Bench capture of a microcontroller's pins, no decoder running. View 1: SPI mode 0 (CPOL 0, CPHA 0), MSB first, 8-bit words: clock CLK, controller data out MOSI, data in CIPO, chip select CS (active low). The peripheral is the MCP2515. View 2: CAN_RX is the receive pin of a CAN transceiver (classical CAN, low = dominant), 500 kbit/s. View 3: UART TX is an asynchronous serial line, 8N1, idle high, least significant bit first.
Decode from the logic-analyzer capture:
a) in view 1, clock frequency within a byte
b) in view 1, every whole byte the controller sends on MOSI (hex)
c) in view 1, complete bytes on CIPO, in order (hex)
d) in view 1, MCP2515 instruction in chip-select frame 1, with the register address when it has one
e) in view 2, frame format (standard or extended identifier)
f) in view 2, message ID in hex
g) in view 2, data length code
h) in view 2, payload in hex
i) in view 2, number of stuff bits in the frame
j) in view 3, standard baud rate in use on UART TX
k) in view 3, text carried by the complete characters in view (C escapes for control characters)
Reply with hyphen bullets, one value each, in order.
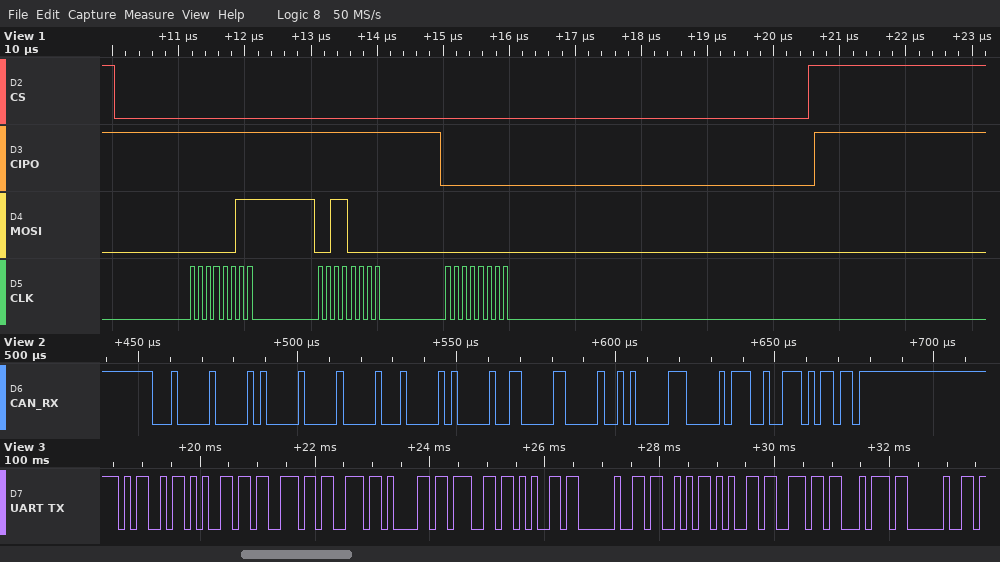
- 8 MHz
- 0x03 0x30 0x00
- 0xFF 0xFF 0x00
- READ 0x30
- standard
- 0x100
- 8
- 00 01 02 03 04 05 06 07
- 11
- 9600 baud
- "Message Sent "
